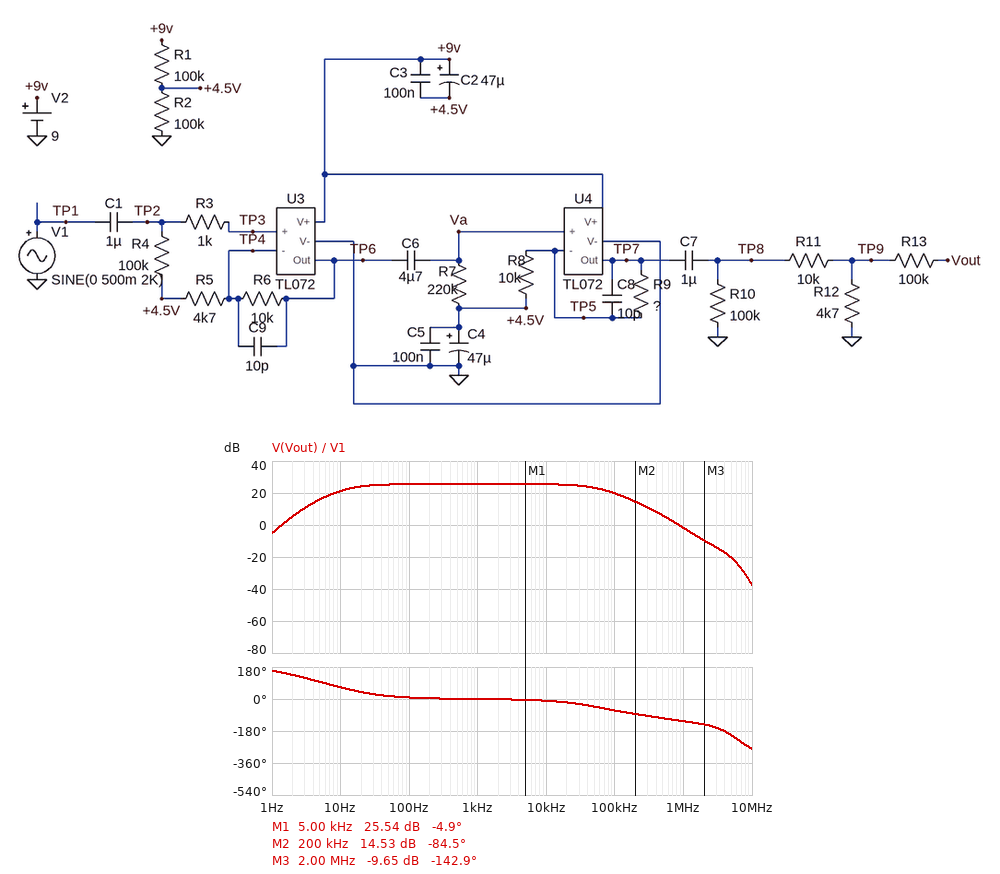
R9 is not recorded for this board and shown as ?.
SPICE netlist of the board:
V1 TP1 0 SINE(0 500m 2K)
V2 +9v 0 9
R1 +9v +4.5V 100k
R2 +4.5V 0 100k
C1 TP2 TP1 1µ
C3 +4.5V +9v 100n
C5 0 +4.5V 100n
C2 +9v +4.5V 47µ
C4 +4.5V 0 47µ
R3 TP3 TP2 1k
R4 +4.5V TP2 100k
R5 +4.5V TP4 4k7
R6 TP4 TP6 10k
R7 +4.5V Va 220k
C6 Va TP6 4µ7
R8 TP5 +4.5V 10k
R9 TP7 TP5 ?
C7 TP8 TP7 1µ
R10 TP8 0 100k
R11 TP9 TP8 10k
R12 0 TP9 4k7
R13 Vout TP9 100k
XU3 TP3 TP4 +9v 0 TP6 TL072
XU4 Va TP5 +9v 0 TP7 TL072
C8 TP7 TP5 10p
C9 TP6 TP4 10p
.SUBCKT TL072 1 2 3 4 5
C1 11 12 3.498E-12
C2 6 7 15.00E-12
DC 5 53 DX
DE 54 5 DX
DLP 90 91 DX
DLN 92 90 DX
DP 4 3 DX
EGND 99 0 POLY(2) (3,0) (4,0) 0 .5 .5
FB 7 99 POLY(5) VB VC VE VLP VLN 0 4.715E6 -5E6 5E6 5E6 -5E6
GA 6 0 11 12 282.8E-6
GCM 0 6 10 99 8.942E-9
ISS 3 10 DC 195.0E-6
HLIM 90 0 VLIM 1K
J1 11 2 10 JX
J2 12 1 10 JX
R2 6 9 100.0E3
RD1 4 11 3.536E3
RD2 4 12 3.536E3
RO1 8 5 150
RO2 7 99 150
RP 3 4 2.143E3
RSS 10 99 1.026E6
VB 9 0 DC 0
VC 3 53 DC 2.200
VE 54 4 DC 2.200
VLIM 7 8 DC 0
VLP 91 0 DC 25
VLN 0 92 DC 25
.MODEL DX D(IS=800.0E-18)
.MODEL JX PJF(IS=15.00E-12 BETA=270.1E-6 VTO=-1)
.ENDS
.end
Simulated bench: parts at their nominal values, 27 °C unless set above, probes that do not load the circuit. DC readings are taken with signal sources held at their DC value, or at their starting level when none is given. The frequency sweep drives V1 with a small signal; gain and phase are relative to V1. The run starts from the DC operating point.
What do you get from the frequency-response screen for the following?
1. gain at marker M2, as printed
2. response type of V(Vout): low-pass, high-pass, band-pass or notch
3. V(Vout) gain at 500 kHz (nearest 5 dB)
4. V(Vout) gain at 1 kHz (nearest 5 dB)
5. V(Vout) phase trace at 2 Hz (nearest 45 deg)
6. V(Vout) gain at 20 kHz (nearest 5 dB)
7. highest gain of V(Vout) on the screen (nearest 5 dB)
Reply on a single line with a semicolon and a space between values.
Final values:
14.53 dB; band-pass; 5 dB; 25 dB; 135 deg; 25 dB; 25 dB
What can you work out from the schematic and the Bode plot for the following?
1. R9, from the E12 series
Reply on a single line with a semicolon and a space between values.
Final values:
180 kΩ
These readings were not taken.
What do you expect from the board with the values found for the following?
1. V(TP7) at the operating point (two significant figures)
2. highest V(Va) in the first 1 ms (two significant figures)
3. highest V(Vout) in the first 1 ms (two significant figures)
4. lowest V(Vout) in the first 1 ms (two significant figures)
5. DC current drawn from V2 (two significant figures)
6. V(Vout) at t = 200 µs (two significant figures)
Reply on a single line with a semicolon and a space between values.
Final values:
4.5 V; 6.1 V; 950 mV; -970 mV; 8.8 mA; 940 mV
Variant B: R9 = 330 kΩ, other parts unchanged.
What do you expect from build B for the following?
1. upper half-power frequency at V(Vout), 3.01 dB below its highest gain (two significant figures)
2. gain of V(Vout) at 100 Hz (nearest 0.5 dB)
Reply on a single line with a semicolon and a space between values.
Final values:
33 kHz; 30.5 dB
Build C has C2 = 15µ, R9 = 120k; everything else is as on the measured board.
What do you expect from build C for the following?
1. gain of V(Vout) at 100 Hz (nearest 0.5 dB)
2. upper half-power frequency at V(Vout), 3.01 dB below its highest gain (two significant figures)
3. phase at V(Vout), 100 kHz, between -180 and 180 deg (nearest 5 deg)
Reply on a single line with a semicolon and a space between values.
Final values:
22.0 dB; 89 kHz; -55 deg
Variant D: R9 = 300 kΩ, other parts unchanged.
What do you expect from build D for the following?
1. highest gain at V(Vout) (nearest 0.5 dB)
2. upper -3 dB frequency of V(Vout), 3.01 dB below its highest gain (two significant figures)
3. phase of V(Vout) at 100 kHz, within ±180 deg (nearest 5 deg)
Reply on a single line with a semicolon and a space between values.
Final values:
30.0 dB; 36 kHz; -75 deg
